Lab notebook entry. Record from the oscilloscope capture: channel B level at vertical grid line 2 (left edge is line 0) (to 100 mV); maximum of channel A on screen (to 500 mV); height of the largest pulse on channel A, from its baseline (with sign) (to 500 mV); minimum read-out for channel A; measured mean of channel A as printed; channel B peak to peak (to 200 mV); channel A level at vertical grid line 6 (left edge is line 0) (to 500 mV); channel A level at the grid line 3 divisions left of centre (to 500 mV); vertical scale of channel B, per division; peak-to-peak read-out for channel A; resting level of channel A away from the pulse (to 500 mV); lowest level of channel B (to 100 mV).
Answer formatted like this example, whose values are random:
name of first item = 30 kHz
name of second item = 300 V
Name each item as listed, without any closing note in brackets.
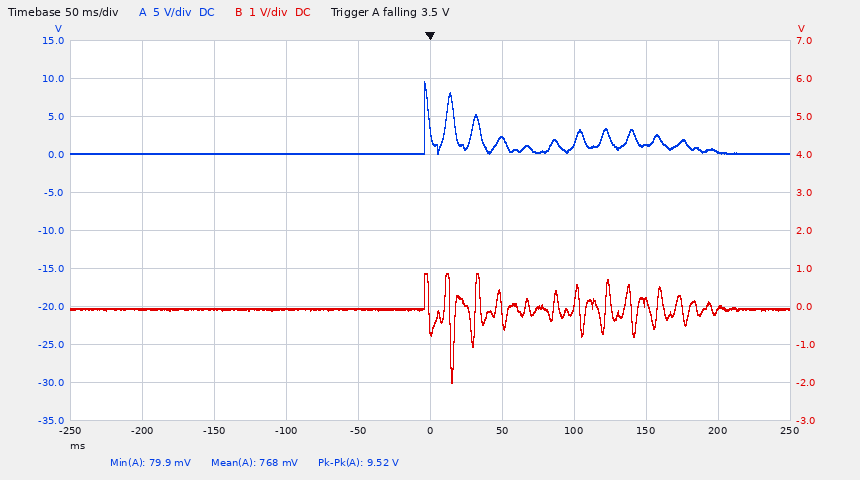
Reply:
channel B level at vertical grid line 2 (left edge is line 0) = -100 mV
maximum of channel A on screen = 9.5 V
height of the largest pulse on channel A, from its baseline (with sign) = +9.5 V
minimum read-out for channel A = 79.9 mV
measured mean of channel A as printed = 768 mV
channel B peak to peak = 2.8 V
channel A level at vertical grid line 6 (left edge is line 0) = 2.0 V
channel A level at the grid line 3 divisions left of centre = 0.0 V
vertical scale of channel B, per division = 1 V
peak-to-peak read-out for channel A = 9.52 V
resting level of channel A away from the pulse = 0.0 V
lowest level of channel B = -2.0 V
